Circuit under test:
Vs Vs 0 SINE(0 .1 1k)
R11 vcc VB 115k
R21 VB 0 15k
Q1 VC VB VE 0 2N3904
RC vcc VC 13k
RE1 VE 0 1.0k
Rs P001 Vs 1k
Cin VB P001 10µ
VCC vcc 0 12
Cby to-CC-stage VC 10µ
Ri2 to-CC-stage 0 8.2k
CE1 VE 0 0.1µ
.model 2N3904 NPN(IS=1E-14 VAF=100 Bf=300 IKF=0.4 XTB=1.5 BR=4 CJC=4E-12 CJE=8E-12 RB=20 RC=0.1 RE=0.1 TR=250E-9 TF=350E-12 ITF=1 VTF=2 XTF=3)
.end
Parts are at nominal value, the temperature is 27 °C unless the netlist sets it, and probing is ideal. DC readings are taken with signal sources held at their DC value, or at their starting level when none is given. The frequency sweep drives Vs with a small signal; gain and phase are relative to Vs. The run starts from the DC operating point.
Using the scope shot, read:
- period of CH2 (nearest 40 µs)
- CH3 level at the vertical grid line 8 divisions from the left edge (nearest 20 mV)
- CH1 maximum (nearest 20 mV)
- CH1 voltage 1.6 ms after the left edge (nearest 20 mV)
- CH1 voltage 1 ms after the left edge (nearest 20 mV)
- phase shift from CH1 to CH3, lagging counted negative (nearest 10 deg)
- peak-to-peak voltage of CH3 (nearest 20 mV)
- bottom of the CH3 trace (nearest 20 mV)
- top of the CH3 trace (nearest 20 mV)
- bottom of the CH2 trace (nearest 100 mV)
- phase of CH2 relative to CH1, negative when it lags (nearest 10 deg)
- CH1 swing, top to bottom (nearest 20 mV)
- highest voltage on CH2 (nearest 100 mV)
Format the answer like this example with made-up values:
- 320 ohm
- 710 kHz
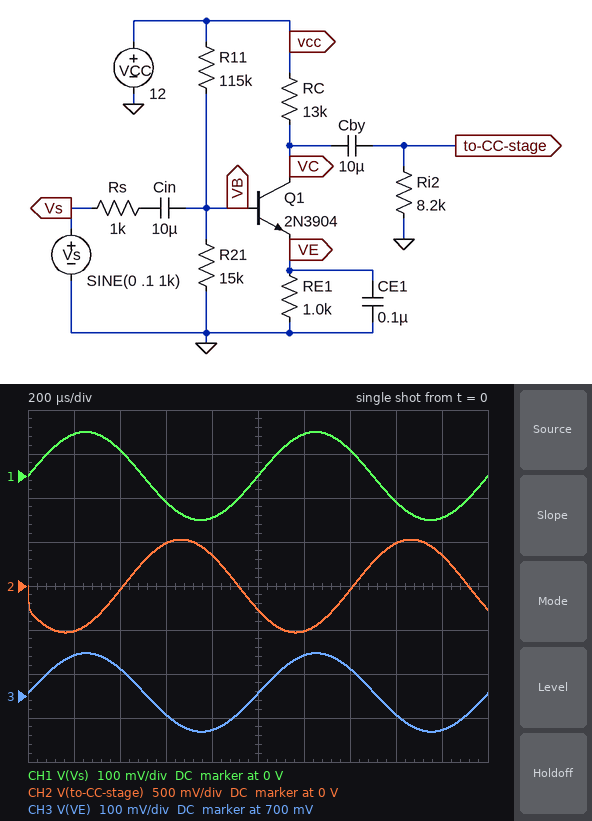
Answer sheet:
- 1.00 ms
- 660 mV
- 100 mV
- -60 mV
- 0 V
- 0 deg
- 180 mV
- 620 mV
- 800 mV
- -500 mV
- -150 deg
- 200 mV
- 500 mV
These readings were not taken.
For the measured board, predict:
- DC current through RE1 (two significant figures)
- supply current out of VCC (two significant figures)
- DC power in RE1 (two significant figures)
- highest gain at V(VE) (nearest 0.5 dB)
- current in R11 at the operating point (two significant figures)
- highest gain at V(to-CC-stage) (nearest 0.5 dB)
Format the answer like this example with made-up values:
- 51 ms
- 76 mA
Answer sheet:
- 710 µA
- 800 µA
- 500 µW
- -1.0 dB
- 93 µA
- 41.0 dB
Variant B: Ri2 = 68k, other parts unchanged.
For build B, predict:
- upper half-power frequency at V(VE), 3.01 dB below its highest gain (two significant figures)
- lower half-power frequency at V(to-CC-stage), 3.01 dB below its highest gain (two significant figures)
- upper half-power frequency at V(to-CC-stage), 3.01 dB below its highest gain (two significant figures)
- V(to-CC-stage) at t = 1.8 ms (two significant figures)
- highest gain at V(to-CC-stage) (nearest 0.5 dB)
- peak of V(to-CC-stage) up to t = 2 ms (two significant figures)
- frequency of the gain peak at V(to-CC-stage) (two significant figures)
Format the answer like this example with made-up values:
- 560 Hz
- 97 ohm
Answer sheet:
- 46 kHz
- 33 kHz
- 260 kHz
- 760 mV
- 47.5 dB
- 1.1 V
- 92 kHz
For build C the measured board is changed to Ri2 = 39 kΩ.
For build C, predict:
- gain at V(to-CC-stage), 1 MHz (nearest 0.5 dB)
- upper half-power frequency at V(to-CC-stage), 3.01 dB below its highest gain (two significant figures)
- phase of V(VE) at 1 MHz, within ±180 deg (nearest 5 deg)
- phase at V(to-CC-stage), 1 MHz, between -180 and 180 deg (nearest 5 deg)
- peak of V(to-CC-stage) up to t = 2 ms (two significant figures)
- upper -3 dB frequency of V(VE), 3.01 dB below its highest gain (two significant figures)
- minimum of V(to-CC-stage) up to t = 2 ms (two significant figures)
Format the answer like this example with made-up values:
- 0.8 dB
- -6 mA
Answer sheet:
- 34.0 dB
- 280 kHz
- -155 deg
- 105 deg
- 1.0 V
- 45 kHz
- -1.0 V
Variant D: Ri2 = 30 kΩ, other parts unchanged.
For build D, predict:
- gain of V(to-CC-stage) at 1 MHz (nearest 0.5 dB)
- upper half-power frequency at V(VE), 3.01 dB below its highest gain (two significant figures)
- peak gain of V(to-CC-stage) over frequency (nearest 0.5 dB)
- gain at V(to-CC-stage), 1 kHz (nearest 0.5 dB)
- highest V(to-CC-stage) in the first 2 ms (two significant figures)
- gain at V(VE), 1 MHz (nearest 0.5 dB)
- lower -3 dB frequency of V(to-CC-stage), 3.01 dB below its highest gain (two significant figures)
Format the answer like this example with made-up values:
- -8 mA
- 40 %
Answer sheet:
- 34.0 dB
- 45 kHz
- 46.0 dB
- 19.5 dB
- 950 mV
- -41.0 dB
- 34 kHz
